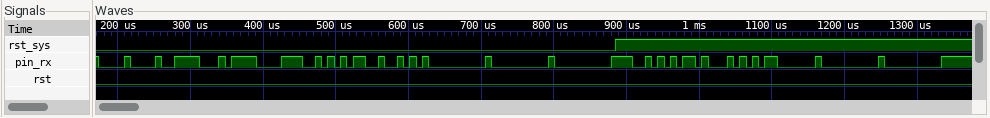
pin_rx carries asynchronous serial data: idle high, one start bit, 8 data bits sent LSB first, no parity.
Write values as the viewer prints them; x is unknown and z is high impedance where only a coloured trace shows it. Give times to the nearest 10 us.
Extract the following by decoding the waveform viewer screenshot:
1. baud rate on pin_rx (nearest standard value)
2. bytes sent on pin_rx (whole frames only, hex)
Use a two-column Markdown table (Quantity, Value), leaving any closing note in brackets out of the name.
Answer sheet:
| Quantity | Value |
|---|---|
| baud rate on pin_rx | 115200 baud |
| bytes sent on pin_rx | 08, 1E, 0F, AA, 52, 00, 00, 00, AA, 51, 03, 00, 00 |
